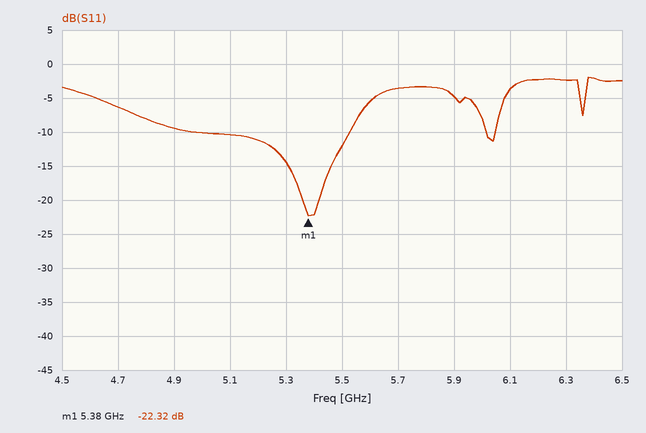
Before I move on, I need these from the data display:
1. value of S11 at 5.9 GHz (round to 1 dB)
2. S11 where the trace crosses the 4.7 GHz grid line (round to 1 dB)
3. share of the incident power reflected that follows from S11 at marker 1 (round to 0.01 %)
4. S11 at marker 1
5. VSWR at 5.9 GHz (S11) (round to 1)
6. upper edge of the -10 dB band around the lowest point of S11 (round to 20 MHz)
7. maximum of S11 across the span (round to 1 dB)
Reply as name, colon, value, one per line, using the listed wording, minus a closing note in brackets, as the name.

value of S11 at 5.9 GHz: -5 dB
S11 where the trace crosses the 4.7 GHz grid line: -6 dB
share of the incident power reflected that follows from S11 at marker 1: 0.59 %
S11 at marker 1: -22.32 dB
VSWR at 5.9 GHz (S11): 4
upper edge of the -10 dB band around the lowest point of S11: 5.52 GHz
maximum of S11 across the span: -2 dB
